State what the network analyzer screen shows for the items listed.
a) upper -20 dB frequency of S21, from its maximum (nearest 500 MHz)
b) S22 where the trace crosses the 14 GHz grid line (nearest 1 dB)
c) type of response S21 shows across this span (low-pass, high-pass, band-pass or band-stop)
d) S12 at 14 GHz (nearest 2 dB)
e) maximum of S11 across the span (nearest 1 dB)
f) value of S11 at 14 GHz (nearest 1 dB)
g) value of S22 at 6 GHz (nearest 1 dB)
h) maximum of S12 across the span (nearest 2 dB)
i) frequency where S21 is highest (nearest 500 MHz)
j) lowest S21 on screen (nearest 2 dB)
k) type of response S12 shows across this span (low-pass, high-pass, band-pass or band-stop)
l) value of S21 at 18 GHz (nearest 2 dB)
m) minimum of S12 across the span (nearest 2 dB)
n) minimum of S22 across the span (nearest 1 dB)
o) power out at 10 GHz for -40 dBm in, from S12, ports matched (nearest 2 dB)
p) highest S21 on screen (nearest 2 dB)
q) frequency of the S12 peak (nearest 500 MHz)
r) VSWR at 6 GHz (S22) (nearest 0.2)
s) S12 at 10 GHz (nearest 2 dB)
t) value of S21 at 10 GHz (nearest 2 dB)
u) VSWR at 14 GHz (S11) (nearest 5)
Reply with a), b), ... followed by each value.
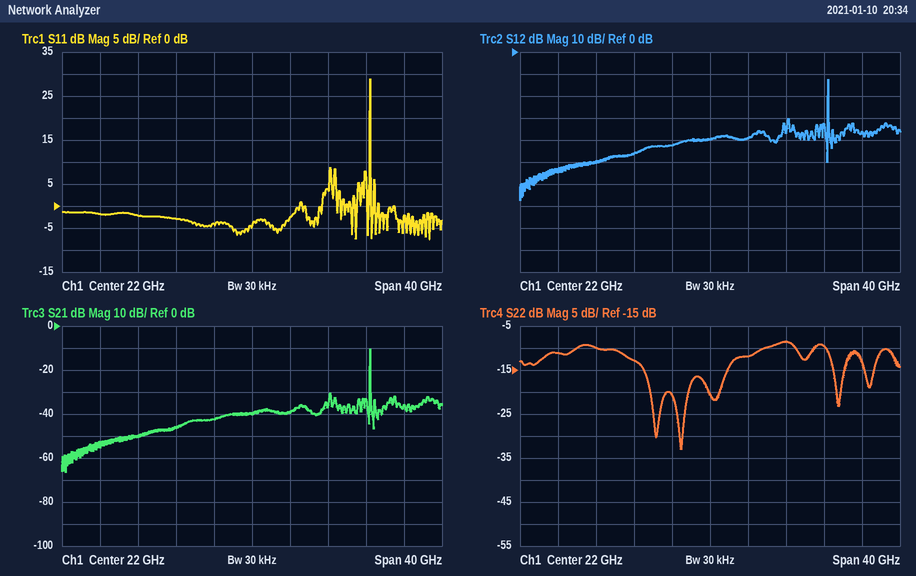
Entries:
a) 34.5 GHz
b) -13 dB
c) band-pass
d) -46 dB
e) 29 dB
f) -3 dB
g) -11 dB
h) -12 dB
i) 34.5 GHz
j) -66 dB
k) band-pass
l) -42 dB
m) -68 dB
n) -33 dB
o) -90 dBm
p) -10 dB
q) 34.5 GHz
r) 1.8
s) -50 dB
t) -50 dB
u) 5
